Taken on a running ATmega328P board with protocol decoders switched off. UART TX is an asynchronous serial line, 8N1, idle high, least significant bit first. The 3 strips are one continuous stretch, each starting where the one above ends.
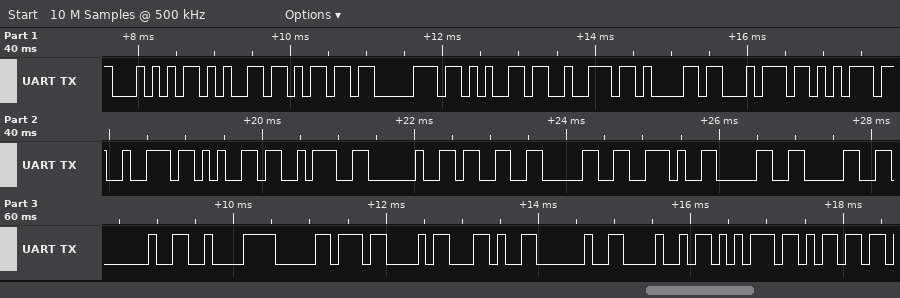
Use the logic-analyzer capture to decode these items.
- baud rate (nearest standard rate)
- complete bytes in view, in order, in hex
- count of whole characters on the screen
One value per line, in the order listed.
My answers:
9600 baud
54 65 6D 70 65 72 61 74 75 72 65 3A 20 33 30 2E 30 30 20 C2 B0 43 2C 20 48 75 6D
27
